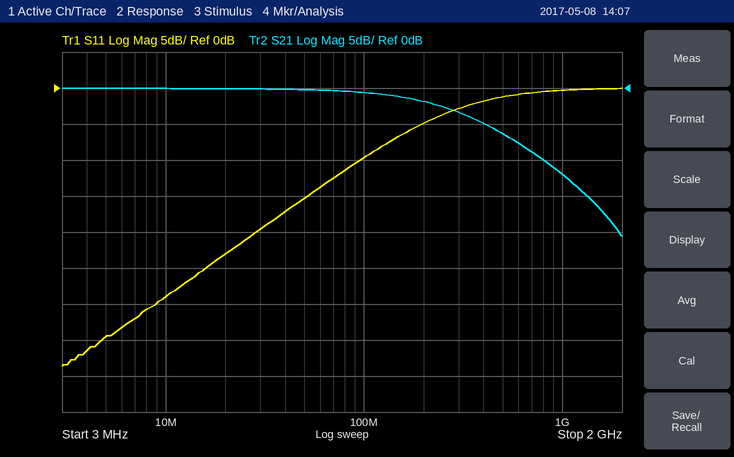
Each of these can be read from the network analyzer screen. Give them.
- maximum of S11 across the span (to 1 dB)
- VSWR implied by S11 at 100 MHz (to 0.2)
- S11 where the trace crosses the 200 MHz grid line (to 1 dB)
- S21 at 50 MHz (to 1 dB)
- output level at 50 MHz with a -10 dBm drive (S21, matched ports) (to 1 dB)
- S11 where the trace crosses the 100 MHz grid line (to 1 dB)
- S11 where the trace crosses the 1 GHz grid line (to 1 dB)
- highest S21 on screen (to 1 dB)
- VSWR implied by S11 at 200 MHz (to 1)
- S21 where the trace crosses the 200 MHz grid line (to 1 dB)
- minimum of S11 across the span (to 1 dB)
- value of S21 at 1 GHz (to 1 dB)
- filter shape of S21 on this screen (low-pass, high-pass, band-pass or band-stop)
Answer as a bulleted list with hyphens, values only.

- 0 dB
- 2.0
- -5 dB
- 0 dB
- -10 dBm
- -10 dB
- 0 dB
- 0 dB
- 4
- -2 dB
- -39 dB
- -12 dB
- low-pass
